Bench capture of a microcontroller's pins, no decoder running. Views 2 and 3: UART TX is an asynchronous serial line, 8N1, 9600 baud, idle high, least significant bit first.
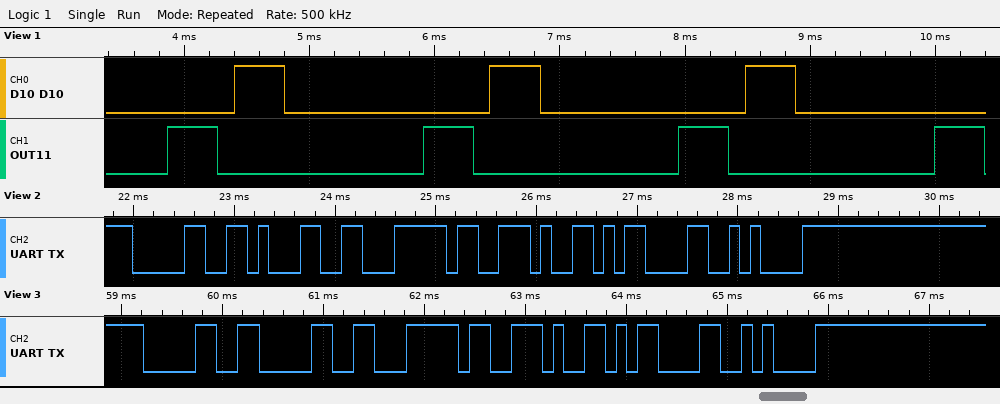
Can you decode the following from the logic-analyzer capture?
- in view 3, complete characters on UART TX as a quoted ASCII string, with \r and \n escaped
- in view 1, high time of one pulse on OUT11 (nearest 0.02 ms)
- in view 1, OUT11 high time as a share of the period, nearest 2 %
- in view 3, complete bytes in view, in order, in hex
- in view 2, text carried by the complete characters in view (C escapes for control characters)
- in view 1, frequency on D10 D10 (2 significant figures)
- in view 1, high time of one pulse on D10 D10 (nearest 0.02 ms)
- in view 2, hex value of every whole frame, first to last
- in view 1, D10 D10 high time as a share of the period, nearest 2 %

"00|.\r\n"
0.40 ms
20 %
0x30 0x30 0x7C 0x2E 0x0D 0x0A
"01|.\r\n"
490 Hz
0.40 ms
30 31 7C 2E 0D 0A
20 %
